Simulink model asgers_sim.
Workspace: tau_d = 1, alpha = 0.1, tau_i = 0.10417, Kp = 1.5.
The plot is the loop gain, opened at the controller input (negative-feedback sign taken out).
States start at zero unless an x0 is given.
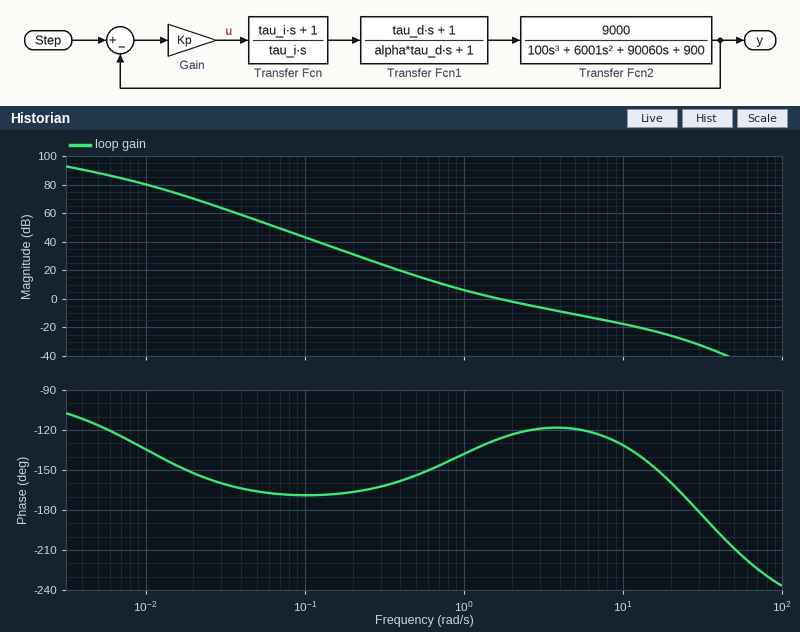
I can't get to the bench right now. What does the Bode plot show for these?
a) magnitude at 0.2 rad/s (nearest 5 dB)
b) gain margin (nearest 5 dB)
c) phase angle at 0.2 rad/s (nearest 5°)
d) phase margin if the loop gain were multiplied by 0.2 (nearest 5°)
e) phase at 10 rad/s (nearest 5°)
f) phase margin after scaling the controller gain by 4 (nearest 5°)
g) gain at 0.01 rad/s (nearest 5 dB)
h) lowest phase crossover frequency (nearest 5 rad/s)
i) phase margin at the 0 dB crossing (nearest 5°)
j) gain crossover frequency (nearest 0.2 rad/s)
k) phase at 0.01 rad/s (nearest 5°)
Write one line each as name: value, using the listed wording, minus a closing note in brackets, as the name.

magnitude at 0.2 rad/s: 30 dB
gain margin: 30 dB
phase angle at 0.2 rad/s: -165°
phase margin if the loop gain were multiplied by 0.2: 30°
phase at 10 rad/s: -130°
phase margin after scaling the controller gain by 4: 60°
gain at 0.01 rad/s: 80 dB
lowest phase crossover frequency: 30 rad/s
phase margin at the 0 dB crossing: 55°
gain crossover frequency: 1.6 rad/s
phase at 0.01 rad/s: -135°
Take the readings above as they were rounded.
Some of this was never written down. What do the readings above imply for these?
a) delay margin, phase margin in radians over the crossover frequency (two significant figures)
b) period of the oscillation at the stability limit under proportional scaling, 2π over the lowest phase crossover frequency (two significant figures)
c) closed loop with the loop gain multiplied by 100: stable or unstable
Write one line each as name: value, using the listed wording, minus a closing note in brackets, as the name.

delay margin, phase margin in radians over the crossover frequency: 0.60 s
period of the oscillation at the stability limit under proportional scaling, 2π over the lowest phase crossover frequency: 0.21 s
closed loop with the loop gain multiplied by 100: stable or unstable: unstable
